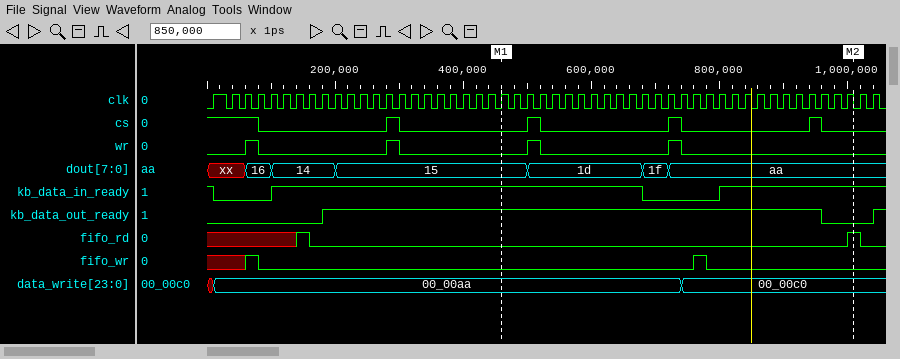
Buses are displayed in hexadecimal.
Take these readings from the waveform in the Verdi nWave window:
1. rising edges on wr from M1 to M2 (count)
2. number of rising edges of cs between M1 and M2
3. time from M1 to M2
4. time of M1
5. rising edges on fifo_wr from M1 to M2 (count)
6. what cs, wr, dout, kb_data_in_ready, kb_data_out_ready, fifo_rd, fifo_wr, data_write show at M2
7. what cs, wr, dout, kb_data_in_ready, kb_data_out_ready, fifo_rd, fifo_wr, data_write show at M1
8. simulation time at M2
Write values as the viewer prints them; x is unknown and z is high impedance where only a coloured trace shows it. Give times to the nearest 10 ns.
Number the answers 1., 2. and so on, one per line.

1. 2
2. 3
3. 550 ns
4. 460 ns
5. 1
6. cs=0, wr=0, dout=aa, kb_data_in_ready=1, kb_data_out_ready=0, fifo_rd=1, fifo_wr=0, data_write=00_00c0
7. cs=0, wr=0, dout=15, kb_data_in_ready=1, kb_data_out_ready=1, fifo_rd=0, fifo_wr=0, data_write=00_00aa
8. 1010 ns
